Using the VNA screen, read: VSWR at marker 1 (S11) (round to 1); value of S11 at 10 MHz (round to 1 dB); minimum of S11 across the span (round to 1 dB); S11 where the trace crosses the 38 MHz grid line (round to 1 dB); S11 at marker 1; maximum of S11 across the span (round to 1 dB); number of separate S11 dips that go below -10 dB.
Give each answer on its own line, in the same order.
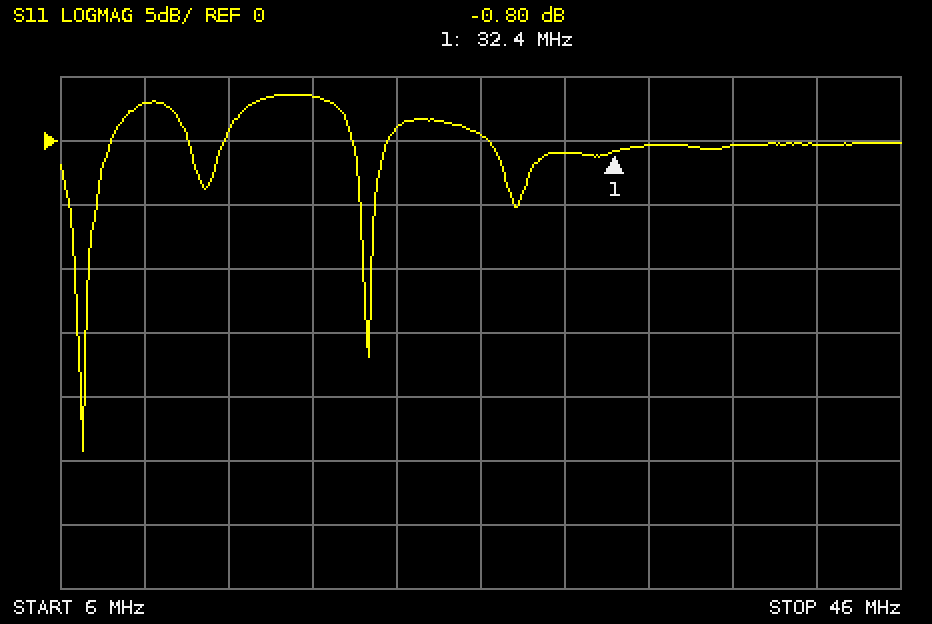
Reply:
22
3 dB
-24 dB
0 dB
-0.80 dB
4 dB
2
